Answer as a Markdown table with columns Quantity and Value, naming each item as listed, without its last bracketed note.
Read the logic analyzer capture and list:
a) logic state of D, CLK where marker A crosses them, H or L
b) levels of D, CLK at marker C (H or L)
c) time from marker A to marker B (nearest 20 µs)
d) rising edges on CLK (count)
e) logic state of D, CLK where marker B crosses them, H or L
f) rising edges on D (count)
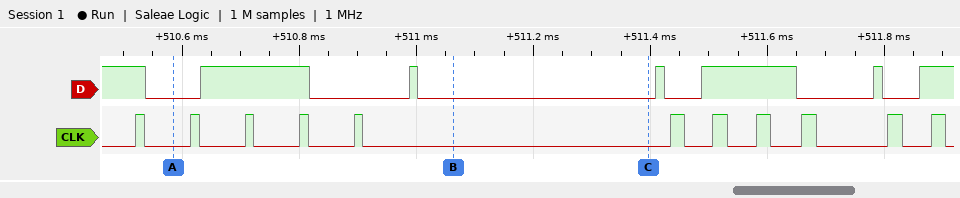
| Quantity | Value |
|---|---|
| logic state of D, CLK where marker A crosses them, H or L | D=L, CLK=L |
| levels of D, CLK at marker C | D=L, CLK=L |
| time from marker A to marker B | 480 µs |
| rising edges on CLK | 11 |
| logic state of D, CLK where marker B crosses them, H or L | D=L, CLK=L |
| rising edges on D | 6 |
